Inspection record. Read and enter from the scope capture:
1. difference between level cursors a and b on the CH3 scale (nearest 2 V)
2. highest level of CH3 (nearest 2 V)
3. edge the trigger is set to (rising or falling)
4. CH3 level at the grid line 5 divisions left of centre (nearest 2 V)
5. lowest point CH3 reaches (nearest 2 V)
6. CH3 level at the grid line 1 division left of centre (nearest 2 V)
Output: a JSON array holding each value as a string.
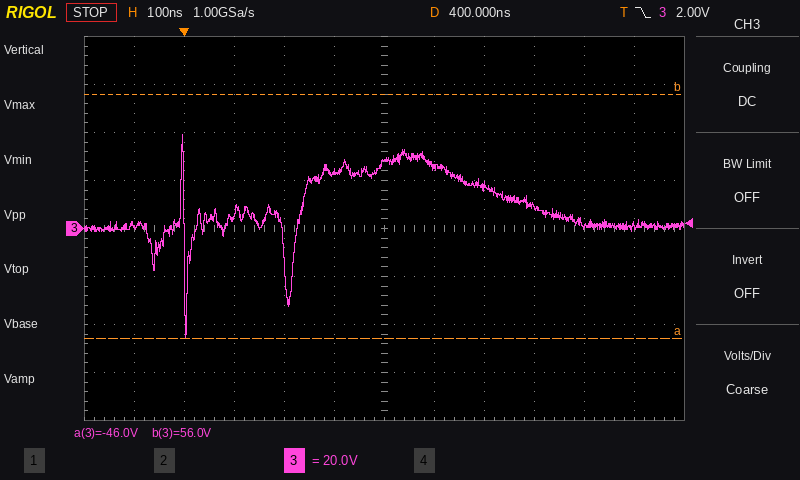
["102 V", "40 V", "falling", "2 V", "-46 V", "24 V"]
